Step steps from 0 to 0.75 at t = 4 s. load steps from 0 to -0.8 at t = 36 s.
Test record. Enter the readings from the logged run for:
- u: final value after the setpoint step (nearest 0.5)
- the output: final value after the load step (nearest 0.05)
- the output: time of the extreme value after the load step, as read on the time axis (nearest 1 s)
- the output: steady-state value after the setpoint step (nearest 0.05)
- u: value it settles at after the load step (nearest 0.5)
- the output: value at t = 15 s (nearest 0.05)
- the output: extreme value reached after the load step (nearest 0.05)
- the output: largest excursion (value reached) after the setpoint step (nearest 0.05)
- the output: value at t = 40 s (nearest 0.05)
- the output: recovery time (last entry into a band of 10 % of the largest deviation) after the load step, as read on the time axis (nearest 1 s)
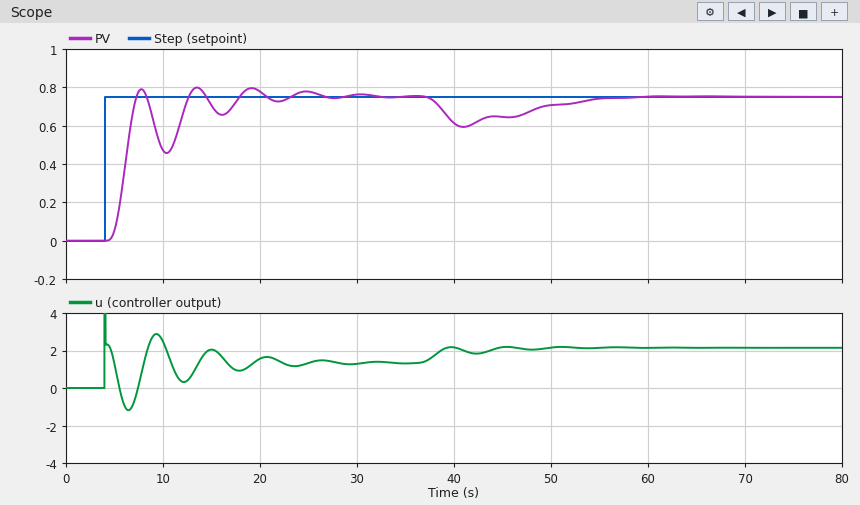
1.5
0.75
41 s
0.75
2.0
0.70
0.60
0.80
0.60
54 s
